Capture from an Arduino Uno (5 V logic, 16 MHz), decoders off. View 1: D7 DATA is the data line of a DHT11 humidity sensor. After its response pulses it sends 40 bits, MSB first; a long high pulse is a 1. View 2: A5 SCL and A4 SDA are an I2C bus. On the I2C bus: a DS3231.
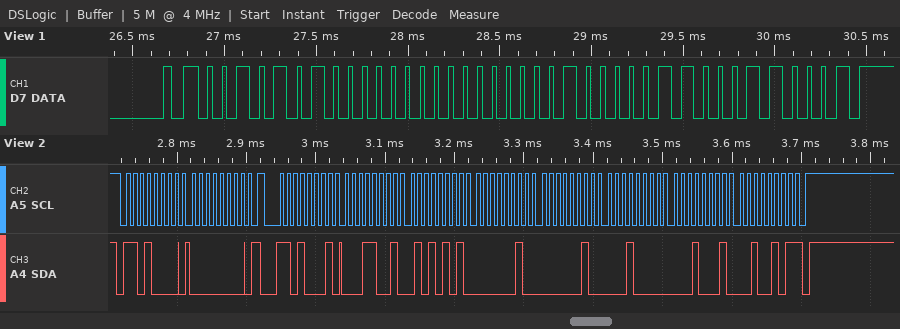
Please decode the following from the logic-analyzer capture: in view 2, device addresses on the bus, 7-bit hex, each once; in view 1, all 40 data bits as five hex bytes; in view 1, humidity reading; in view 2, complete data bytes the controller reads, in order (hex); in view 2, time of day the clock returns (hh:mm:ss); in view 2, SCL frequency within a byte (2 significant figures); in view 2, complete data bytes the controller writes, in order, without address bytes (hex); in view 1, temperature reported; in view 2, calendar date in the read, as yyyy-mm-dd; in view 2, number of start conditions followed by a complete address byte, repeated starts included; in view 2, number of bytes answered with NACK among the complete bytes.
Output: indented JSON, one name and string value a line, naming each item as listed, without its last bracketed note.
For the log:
{
  "in view 2, device addresses on the bus, 7-bit hex, each once": "0x68",
  "in view 1, all 40 data bits as five hex bytes": "2A 00 01 06 31",
  "in view 1, humidity reading": "42 %",
  "in view 2, complete data bytes the controller reads, in order": "19 55 02 02 10 11 25",
  "in view 2, time of day the clock returns": "02:55:19",
  "in view 2, SCL frequency within a byte": "100 kHz",
  "in view 2, complete data bytes the controller writes, in order, without address bytes": "00",
  "in view 1, temperature reported": "1.6 °C",
  "in view 2, calendar date in the read, as yyyy-mm-dd": "2025-11-10",
  "in view 2, number of start conditions followed by a complete address byte, repeated starts included": "2",
  "in view 2, number of bytes answered with NACK among the complete bytes": "1"
}
